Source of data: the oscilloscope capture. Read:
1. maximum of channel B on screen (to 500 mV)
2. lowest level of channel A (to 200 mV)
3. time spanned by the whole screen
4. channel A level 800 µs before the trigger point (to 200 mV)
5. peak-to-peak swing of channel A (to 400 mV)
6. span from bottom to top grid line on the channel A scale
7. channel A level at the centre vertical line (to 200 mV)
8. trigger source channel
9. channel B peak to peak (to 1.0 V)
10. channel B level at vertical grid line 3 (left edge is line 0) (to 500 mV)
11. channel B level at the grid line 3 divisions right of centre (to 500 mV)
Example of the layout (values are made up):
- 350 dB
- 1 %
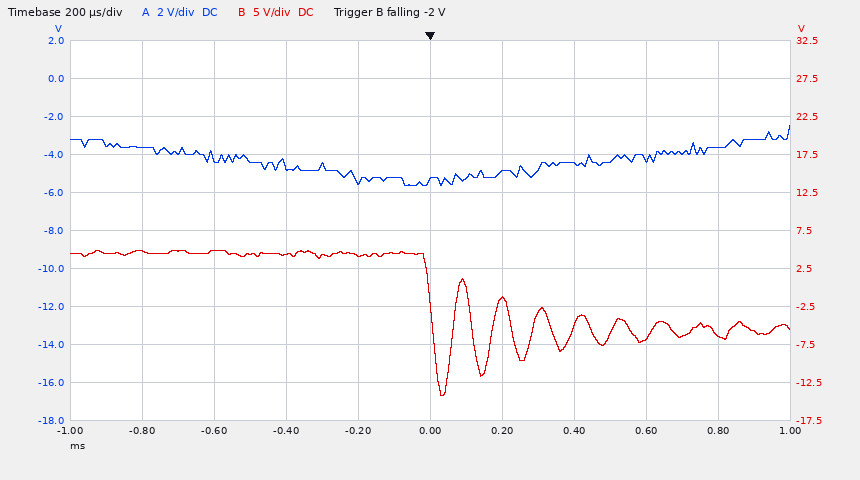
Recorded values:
- 5.0 V
- -5.6 V
- 2 ms
- -3.6 V
- 3.2 V
- 20 V
- -5.4 V
- channel B
- 19.0 V
- 4.5 V
- -6.5 V
